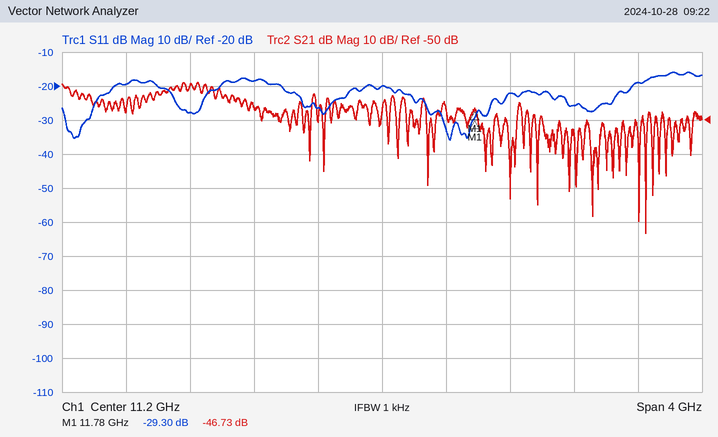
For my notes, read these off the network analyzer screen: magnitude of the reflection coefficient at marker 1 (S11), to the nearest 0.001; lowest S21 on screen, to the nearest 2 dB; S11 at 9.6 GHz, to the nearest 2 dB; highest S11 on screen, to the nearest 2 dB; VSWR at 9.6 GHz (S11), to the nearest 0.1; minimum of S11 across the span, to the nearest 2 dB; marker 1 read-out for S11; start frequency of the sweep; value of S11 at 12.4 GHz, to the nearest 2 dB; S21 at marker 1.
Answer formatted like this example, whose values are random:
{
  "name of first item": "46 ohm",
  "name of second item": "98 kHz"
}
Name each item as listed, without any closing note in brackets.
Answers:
{
  "magnitude of the reflection coefficient at marker 1 (S11), to the nearest 0.001": "0.034",
  "lowest S21 on screen, to the nearest 2 dB": "-84 dB",
  "S11 at 9.6 GHz, to the nearest 2 dB": "-20 dB",
  "highest S11 on screen, to the nearest 2 dB": "-16 dB",
  "VSWR at 9.6 GHz (S11), to the nearest 0.1": "1.2",
  "minimum of S11 across the span, to the nearest 2 dB": "-36 dB",
  "marker 1 read-out for S11": "-29.30 dB",
  "start frequency of the sweep": "9.2 GHz",
  "value of S11 at 12.4 GHz, to the nearest 2 dB": "-26 dB",
  "S21 at marker 1": "-46.73 dB"
}
